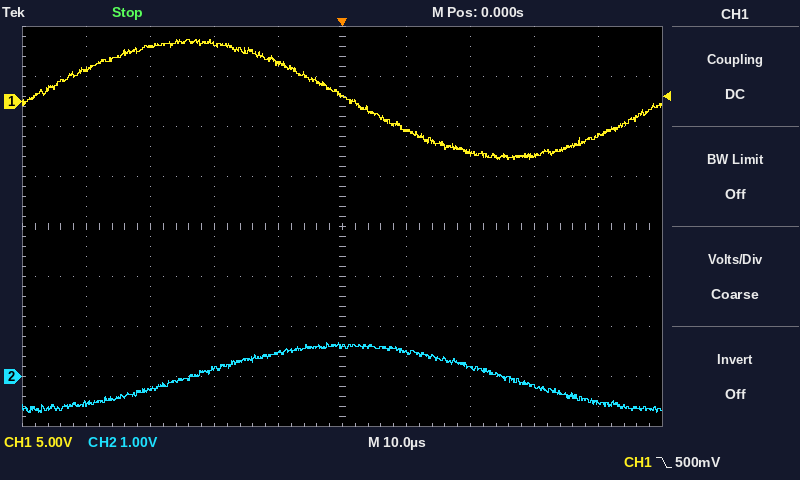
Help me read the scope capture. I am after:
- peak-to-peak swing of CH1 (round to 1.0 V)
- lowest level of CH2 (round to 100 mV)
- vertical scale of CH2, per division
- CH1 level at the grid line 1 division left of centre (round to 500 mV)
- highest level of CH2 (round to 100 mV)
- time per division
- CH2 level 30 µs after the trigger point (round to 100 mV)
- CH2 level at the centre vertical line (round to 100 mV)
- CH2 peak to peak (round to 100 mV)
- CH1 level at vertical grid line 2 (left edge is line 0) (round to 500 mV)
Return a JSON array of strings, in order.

["12.0 V", "-700 mV", "1 V", "4.0 V", "700 mV", "10 µs", "-200 mV", "600 mV", "1.4 V", "5.5 V"]
